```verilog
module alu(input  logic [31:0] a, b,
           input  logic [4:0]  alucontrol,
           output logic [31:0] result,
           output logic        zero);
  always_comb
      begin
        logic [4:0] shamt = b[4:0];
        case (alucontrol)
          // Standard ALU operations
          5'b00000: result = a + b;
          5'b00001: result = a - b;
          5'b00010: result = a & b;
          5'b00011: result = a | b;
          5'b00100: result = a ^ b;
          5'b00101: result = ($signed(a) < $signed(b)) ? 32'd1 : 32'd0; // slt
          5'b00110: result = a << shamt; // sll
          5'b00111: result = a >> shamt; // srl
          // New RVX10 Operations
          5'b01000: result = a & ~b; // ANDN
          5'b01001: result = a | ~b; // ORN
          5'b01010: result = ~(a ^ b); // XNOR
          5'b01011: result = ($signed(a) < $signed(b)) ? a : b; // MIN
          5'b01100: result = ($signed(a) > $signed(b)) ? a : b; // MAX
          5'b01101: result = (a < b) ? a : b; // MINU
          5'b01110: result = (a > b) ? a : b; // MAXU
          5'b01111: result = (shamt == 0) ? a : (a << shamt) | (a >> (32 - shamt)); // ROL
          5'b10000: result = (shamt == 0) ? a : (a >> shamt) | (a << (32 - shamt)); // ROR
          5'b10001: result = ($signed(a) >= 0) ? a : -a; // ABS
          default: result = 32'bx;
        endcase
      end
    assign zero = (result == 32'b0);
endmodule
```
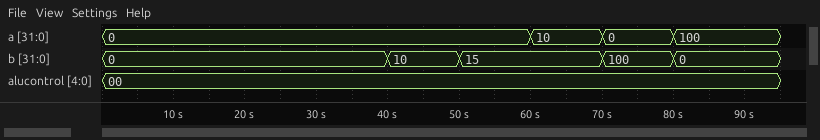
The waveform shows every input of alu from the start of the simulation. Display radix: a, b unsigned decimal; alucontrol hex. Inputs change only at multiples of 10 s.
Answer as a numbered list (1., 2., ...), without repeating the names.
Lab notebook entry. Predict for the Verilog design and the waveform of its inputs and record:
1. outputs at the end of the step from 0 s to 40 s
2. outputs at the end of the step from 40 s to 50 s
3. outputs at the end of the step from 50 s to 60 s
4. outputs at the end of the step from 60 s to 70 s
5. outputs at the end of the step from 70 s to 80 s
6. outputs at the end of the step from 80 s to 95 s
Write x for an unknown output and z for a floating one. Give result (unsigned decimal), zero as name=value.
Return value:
1. result=0, zero=1
2. result=10, zero=0
3. result=15, zero=0
4. result=25, zero=0
5. result=100, zero=0
6. result=100, zero=0
